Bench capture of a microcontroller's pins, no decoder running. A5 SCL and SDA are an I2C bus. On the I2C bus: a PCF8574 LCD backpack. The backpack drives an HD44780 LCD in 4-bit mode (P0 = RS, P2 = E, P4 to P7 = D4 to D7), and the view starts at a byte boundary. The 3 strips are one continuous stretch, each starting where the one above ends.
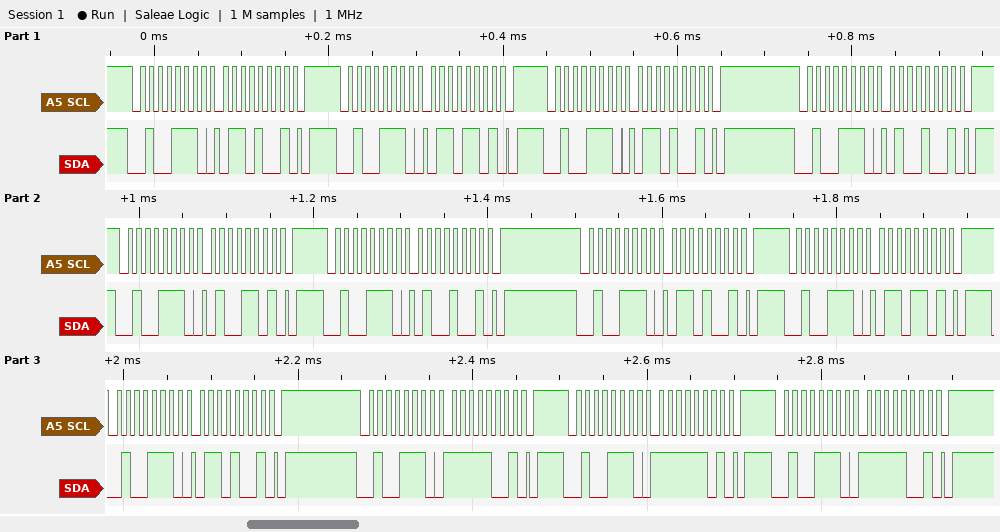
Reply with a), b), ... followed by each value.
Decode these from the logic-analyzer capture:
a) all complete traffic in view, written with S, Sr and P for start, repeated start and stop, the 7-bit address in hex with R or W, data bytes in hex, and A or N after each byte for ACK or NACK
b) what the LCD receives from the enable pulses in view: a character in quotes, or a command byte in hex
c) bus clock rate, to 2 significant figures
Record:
a) S 27W A 69 A P S 27W A 6D A P S 27W A 69 A P S 27W A 49 A P S 27W A 4D A P S 27W A 49 A P S 27W A 69 A P S 27W A 6D A P S 27W A 69 A P S 27W A F9 A P S 27W A FD A P S 27W A F9 A P
b) 'd' 'o'
c) 100 kHz
